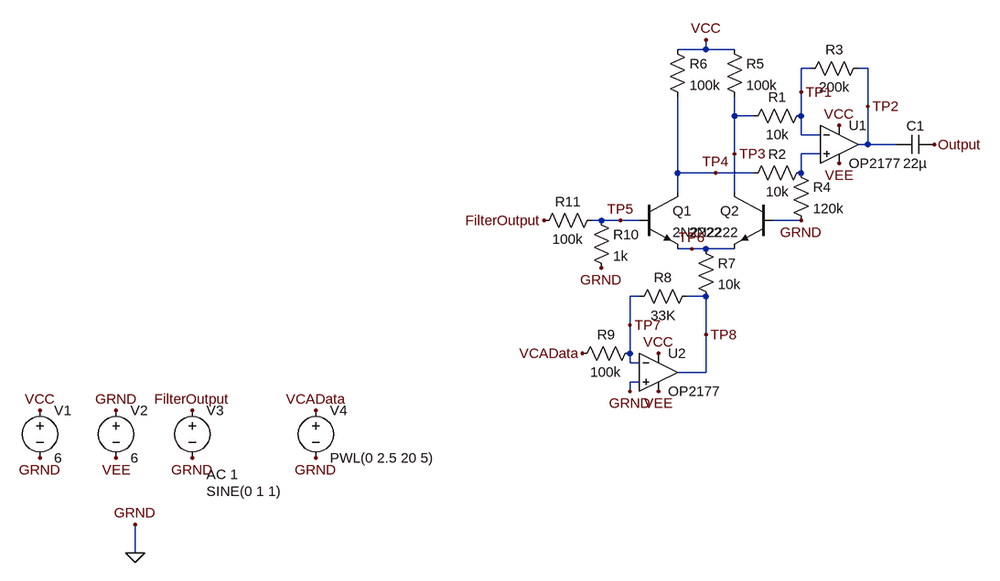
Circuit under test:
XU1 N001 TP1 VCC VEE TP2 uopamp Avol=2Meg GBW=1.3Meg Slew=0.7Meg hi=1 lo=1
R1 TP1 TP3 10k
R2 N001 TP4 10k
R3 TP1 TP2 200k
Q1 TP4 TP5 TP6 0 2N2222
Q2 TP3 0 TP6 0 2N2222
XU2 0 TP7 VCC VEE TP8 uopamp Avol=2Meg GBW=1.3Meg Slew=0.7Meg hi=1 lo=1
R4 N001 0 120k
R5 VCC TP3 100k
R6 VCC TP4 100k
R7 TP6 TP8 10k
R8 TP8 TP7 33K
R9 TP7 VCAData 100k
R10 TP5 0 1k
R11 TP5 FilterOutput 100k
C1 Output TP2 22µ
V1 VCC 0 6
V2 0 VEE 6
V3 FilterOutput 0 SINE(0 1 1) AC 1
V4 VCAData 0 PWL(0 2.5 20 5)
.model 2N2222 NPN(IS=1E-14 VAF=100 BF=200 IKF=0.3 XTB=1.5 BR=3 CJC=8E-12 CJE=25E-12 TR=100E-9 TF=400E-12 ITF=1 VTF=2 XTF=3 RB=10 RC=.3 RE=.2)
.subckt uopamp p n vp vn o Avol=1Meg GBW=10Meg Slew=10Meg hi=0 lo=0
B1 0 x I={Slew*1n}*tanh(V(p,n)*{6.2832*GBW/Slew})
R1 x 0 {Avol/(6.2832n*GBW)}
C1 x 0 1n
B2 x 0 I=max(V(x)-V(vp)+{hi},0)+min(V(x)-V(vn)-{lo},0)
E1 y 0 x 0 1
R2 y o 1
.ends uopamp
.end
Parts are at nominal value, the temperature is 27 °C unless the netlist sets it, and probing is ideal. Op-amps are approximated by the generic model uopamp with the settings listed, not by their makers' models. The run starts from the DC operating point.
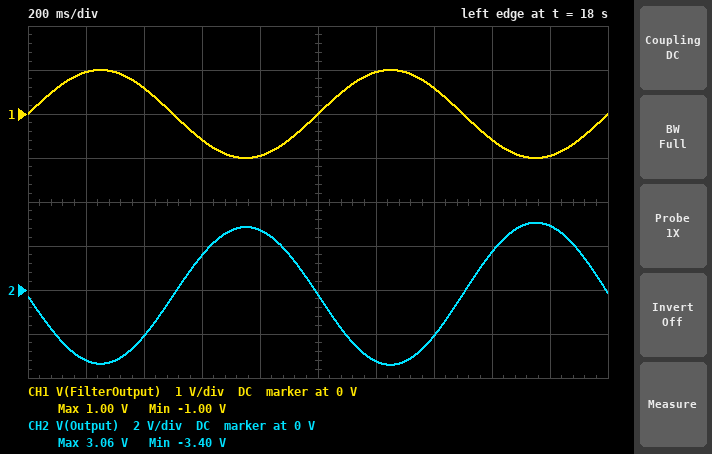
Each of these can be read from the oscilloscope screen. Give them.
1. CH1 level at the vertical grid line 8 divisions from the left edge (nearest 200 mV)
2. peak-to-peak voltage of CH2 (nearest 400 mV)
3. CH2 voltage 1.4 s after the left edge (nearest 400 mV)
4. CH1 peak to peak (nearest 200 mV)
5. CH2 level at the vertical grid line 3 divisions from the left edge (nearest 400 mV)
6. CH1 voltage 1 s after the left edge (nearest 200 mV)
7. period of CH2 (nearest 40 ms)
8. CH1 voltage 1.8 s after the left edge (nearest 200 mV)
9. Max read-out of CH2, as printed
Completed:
-600 mV
6.4 V
-2.0 V
2.0 V
1.6 V
0 V
1.00 s
-1.0 V
3.06 V
